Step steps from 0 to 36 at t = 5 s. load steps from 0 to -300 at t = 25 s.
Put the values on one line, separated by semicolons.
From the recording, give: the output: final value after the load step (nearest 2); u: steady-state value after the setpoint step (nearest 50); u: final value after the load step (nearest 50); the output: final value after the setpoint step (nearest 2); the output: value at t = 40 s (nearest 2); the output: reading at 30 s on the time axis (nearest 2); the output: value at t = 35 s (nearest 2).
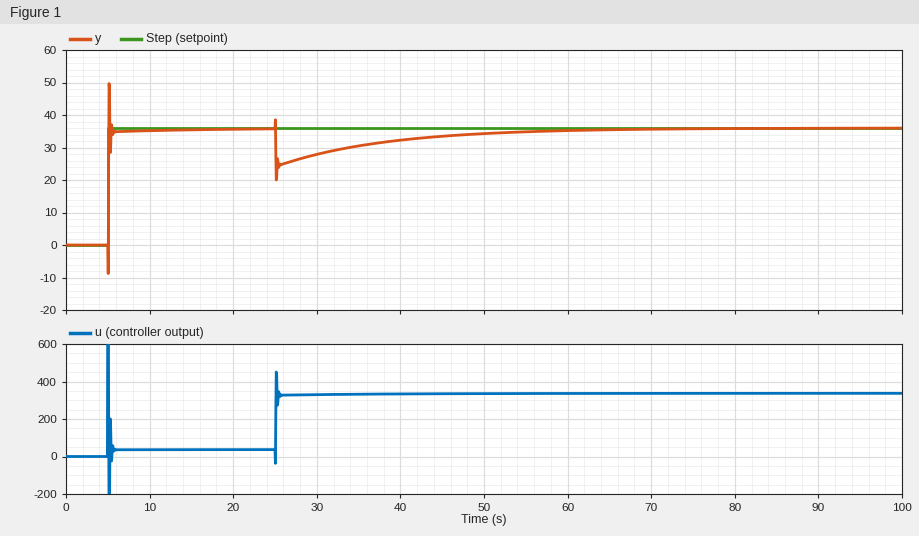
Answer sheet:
36; 50; 350; 36; 32; 28; 30
